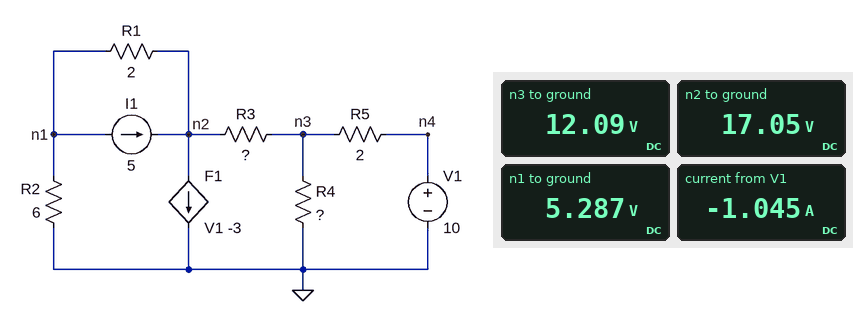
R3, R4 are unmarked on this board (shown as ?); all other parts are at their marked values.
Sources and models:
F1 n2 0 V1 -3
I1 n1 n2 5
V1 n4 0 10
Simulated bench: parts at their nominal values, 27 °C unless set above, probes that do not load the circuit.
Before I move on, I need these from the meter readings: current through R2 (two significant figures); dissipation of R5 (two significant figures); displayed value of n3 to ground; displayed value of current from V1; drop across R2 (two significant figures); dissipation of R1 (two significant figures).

880 mA
2.2 W
12.09 V
-1.045 A
5.3 V
69 W
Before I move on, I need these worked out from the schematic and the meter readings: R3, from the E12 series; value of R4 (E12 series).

2.2 Ω
10 Ω
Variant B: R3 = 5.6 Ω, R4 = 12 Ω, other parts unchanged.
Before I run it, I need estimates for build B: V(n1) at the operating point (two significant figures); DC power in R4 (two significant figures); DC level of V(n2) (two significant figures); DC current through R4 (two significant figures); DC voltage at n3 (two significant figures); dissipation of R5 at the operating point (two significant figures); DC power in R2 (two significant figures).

15 V
16 W
30 V
1.1 A
14 V
6.8 W
39 W
